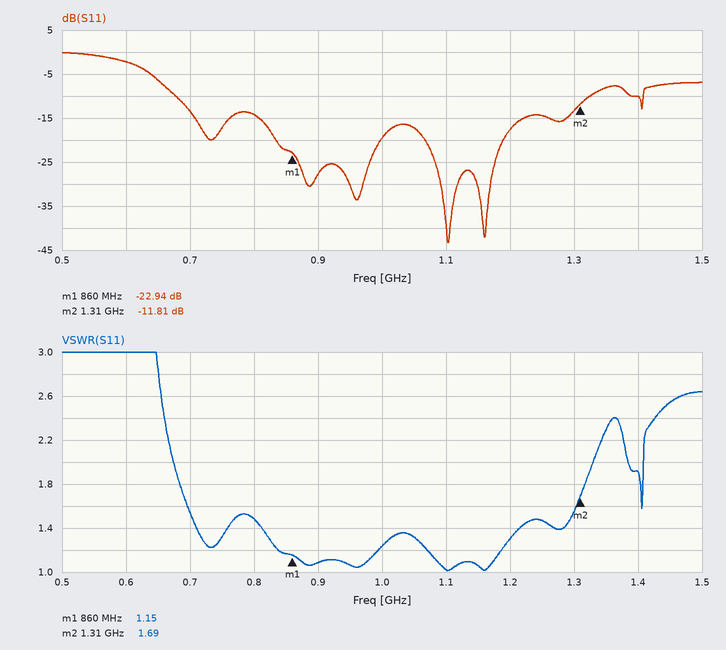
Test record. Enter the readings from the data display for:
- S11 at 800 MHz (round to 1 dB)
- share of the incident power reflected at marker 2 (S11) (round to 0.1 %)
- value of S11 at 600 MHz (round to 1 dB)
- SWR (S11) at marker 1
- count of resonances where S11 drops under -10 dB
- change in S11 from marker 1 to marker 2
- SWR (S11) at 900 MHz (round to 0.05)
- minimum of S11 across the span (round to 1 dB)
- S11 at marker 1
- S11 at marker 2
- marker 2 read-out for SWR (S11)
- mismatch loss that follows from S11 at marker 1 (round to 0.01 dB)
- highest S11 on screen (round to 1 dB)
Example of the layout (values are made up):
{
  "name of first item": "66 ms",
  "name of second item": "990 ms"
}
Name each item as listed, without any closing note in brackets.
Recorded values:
{
  "S11 at 800 MHz": "-14 dB",
  "share of the incident power reflected at marker 2 (S11)": "6.6 %",
  "value of S11 at 600 MHz": "-2 dB",
  "SWR (S11) at marker 1": "1.15",
  "count of resonances where S11 drops under -10 dB": "6",
  "change in S11 from marker 1 to marker 2": "11.13 dB",
  "SWR (S11) at 900 MHz": "1.10",
  "minimum of S11 across the span": "-43 dB",
  "S11 at marker 1": "-22.94 dB",
  "S11 at marker 2": "-11.81 dB",
  "marker 2 read-out for SWR": "1.69",
  "mismatch loss that follows from S11 at marker 1": "0.02 dB",
  "highest S11 on screen": "0 dB"
}
